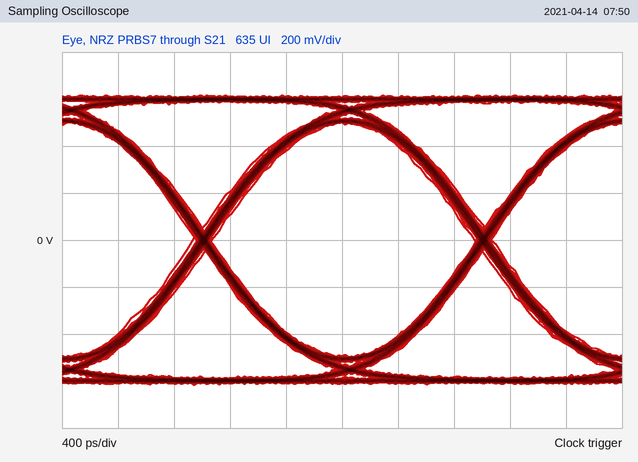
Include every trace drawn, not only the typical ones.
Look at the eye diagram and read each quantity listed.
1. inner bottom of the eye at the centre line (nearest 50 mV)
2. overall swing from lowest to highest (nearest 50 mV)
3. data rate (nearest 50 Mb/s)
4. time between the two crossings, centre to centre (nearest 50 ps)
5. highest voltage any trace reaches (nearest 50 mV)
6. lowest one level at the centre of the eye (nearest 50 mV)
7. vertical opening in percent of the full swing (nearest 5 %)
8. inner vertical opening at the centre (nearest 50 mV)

-500 mV
1.25 V
500 Mb/s
2.00 ns
600 mV
500 mV
80 %
1.00 V
